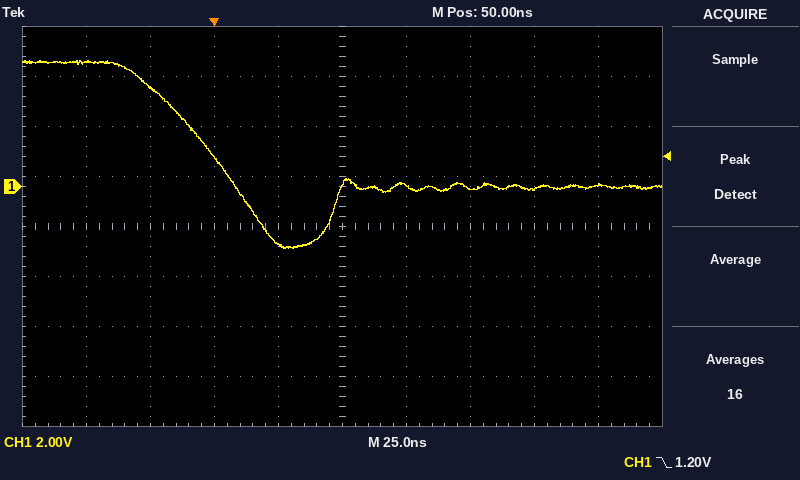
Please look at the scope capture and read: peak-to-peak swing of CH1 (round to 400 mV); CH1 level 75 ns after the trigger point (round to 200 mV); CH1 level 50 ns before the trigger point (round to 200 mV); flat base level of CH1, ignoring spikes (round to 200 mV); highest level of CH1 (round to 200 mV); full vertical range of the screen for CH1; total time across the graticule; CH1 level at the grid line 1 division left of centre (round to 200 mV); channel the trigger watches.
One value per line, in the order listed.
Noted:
7.6 V
0.0 V
5.0 V
0.0 V
5.0 V
16 V
250 ns
-2.4 V
CH1
